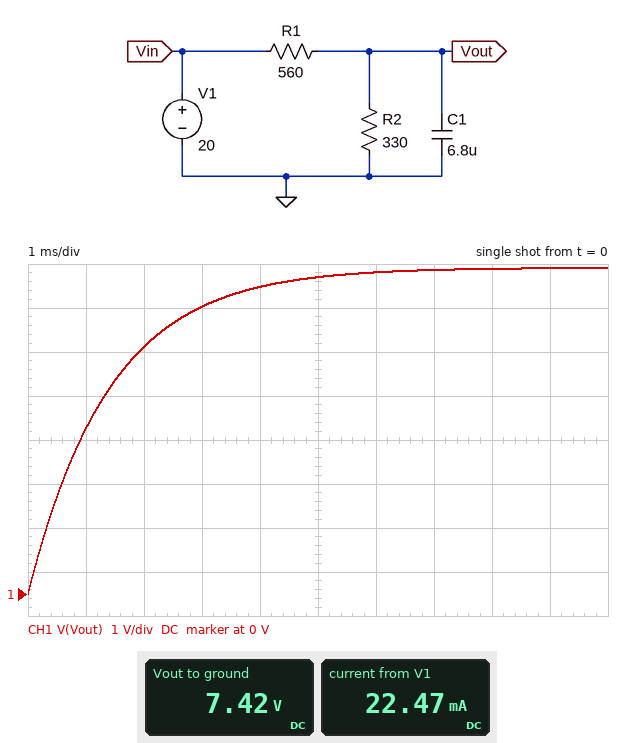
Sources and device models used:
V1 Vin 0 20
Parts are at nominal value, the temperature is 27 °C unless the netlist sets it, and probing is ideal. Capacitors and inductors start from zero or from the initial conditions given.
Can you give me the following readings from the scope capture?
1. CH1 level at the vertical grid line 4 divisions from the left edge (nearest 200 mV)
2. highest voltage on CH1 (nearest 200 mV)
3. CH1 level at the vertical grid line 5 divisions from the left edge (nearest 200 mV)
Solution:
7.0 V
7.4 V
7.2 V
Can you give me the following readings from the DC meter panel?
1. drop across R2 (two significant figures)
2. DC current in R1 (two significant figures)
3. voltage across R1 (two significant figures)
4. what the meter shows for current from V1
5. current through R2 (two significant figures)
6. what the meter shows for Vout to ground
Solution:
7.4 V
22 mA
13 V
22.47 mA
22 mA
7.42 V
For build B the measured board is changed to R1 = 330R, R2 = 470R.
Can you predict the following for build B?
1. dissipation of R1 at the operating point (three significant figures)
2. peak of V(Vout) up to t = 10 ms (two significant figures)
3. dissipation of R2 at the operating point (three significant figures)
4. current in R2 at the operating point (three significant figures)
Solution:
206 mW
12 V
294 mW
25.0 mA
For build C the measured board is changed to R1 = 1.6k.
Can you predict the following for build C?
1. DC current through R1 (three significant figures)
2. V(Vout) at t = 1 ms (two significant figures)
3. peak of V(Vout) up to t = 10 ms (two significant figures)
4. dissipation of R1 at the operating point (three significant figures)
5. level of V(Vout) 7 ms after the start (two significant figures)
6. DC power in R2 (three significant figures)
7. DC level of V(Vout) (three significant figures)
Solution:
10.4 mA
1.4 V
3.4 V
172 mW
3.3 V
35.4 mW
3.42 V
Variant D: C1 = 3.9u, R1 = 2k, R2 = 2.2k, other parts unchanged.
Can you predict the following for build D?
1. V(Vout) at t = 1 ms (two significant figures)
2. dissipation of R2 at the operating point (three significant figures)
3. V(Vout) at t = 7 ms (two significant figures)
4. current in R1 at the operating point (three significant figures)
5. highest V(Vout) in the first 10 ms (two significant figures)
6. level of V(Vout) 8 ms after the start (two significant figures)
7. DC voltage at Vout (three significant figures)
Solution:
2.3 V
49.9 mW
8.6 V
4.76 mA
9.6 V
9.0 V
10.5 V
